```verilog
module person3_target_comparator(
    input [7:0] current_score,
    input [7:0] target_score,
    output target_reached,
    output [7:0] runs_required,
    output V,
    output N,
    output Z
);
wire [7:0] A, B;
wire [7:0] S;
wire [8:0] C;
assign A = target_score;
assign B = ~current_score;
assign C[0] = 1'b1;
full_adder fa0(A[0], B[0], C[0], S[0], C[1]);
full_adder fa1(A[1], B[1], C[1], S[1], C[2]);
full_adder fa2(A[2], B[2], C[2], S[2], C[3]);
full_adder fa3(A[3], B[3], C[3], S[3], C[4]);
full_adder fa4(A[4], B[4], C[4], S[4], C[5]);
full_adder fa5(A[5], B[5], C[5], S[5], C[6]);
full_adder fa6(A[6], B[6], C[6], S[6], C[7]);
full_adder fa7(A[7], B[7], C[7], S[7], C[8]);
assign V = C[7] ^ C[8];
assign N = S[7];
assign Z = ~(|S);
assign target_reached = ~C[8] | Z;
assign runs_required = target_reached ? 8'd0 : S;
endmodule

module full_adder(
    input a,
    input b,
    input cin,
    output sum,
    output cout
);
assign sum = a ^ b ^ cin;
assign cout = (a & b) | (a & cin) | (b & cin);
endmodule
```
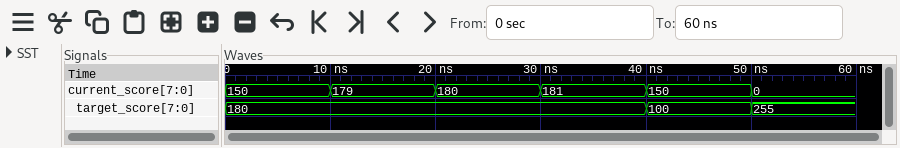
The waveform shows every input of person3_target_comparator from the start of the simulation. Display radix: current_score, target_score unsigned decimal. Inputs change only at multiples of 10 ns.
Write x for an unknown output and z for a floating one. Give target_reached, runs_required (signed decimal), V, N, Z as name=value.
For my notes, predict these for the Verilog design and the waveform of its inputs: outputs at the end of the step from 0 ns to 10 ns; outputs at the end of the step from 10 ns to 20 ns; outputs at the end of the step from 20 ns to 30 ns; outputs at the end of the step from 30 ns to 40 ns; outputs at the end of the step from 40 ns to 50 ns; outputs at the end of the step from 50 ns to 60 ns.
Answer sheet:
target_reached=0, runs_required=30, V=0, N=0, Z=0
target_reached=0, runs_required=1, V=0, N=0, Z=0
target_reached=1, runs_required=0, V=0, N=0, Z=1
target_reached=1, runs_required=0, V=0, N=1, Z=0
target_reached=1, runs_required=0, V=1, N=1, Z=0
target_reached=0, runs_required=-1, V=0, N=1, Z=0
